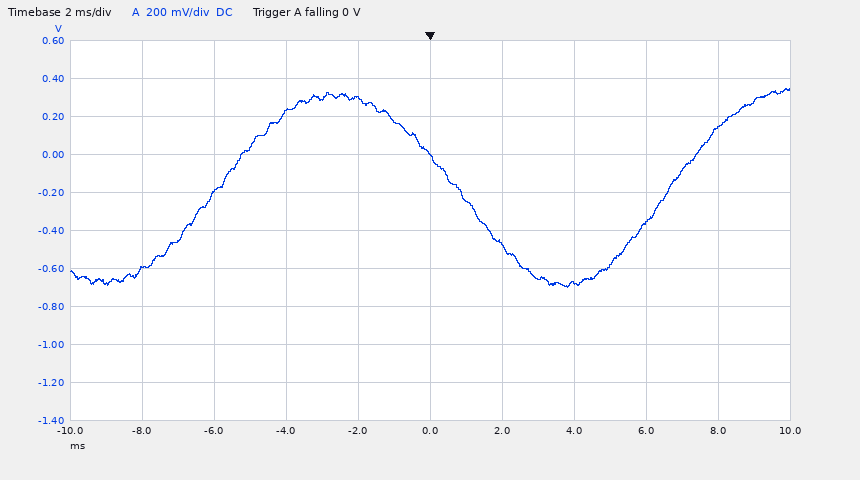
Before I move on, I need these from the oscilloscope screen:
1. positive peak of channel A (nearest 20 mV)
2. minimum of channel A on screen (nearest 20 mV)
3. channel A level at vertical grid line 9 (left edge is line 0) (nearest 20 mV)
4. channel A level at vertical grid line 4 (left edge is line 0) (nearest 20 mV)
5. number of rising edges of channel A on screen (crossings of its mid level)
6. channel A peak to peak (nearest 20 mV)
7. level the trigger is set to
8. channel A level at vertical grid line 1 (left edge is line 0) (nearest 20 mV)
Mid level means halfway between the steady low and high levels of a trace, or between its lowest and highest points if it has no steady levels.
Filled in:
340 mV
-700 mV
140 mV
300 mV
2
1.04 V
0 V
-600 mV
